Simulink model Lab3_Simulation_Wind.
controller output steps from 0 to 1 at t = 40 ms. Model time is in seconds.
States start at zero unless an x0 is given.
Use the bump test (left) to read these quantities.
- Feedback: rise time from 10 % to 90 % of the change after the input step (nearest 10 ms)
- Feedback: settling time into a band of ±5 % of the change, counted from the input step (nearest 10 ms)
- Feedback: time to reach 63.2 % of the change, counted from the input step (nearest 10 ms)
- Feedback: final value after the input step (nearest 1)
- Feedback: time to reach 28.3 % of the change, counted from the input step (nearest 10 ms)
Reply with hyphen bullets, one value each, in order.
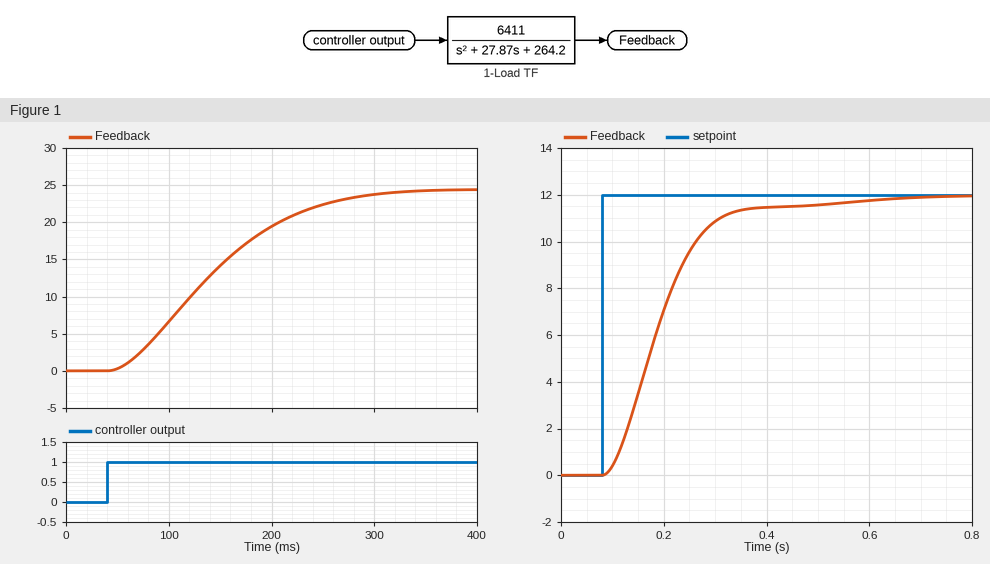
- 170 ms
- 230 ms
- 120 ms
- 24
- 60 ms
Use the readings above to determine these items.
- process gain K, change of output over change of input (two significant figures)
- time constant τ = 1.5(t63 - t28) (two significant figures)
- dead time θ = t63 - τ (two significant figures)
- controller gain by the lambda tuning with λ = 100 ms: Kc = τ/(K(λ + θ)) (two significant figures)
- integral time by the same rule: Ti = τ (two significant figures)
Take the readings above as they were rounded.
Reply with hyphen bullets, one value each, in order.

- 24
- 90 ms
- 30 ms
- 0.029
- 90 ms
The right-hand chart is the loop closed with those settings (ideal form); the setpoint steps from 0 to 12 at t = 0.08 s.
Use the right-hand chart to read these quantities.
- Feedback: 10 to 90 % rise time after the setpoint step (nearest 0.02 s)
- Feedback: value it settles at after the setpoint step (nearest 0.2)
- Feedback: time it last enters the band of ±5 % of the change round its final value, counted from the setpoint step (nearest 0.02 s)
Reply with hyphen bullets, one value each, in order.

- 0.18 s
- 12.0
- 0.28 s
